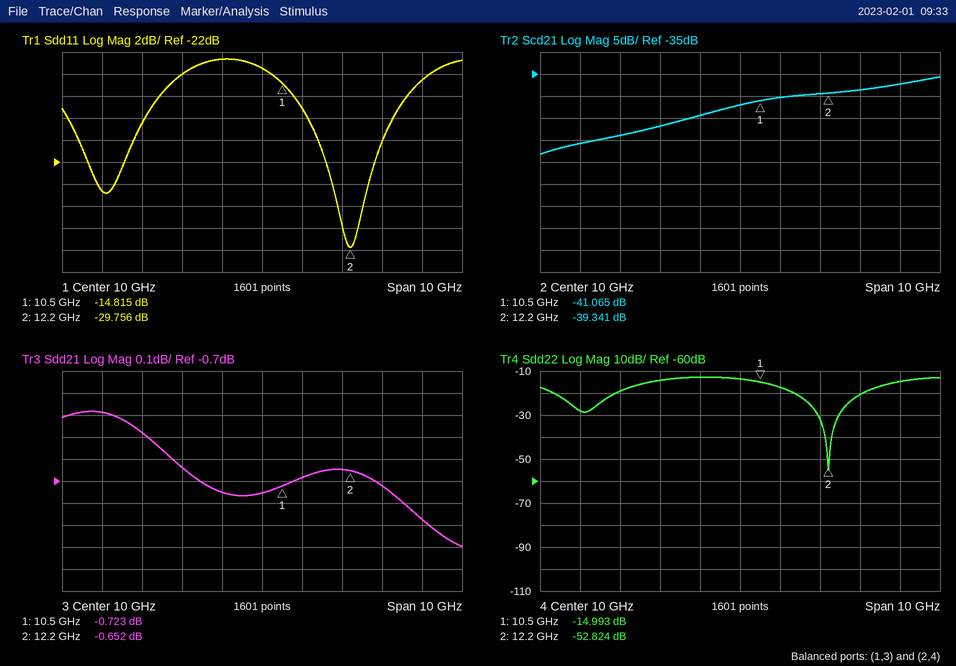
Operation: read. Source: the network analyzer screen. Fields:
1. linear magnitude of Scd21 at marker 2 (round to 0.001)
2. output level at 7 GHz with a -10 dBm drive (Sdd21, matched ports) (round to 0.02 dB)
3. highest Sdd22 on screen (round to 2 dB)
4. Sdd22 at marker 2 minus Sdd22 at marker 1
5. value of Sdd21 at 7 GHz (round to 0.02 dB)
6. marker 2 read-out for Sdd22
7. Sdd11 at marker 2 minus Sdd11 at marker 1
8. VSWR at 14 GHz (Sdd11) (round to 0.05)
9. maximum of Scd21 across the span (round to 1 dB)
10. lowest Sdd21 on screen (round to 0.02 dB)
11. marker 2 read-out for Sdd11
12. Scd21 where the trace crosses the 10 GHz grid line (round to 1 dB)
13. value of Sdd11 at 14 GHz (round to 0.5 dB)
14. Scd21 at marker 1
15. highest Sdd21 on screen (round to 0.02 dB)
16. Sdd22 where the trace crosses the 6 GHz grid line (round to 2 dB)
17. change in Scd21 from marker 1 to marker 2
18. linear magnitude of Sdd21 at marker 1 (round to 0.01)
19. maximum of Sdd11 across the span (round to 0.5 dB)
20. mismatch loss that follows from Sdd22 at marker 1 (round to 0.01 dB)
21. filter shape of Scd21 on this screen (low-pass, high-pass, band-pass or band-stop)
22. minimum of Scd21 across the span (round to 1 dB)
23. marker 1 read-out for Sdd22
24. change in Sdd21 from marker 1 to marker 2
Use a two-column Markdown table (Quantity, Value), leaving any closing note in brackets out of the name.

| Quantity | Value |
|---|---|
| linear magnitude of Scd21 at marker 2 | 0.011 |
| output level at 7 GHz with a -10 dBm drive (Sdd21, matched ports) | -10.48 dBm |
| highest Sdd22 on screen | -12 dB |
| Sdd22 at marker 2 minus Sdd22 at marker 1 | -37.831 dB |
| value of Sdd21 at 7 GHz | -0.48 dB |
| marker 2 read-out for Sdd22 | -52.824 dB |
| Sdd11 at marker 2 minus Sdd11 at marker 1 | -14.941 dB |
| VSWR at 14 GHz (Sdd11) | 1.45 |
| maximum of Scd21 across the span | -36 dB |
| lowest Sdd21 on screen | -1.00 dB |
| marker 2 read-out for Sdd11 | -29.756 dB |
| Scd21 where the trace crosses the 10 GHz grid line | -42 dB |
| value of Sdd11 at 14 GHz | -14.5 dB |
| Scd21 at marker 1 | -41.065 dB |
| highest Sdd21 on screen | -0.38 dB |
| Sdd22 where the trace crosses the 6 GHz grid line | -28 dB |
| change in Scd21 from marker 1 to marker 2 | 1.724 dB |
| linear magnitude of Sdd21 at marker 1 | 0.92 |
| maximum of Sdd11 across the span | -12.5 dB |
| mismatch loss that follows from Sdd22 at marker 1 | 0.14 dB |
| filter shape of Scd21 on this screen | high-pass |
| minimum of Scd21 across the span | -53 dB |
| marker 1 read-out for Sdd22 | -14.993 dB |
| change in Sdd21 from marker 1 to marker 2 | 0.071 dB |
